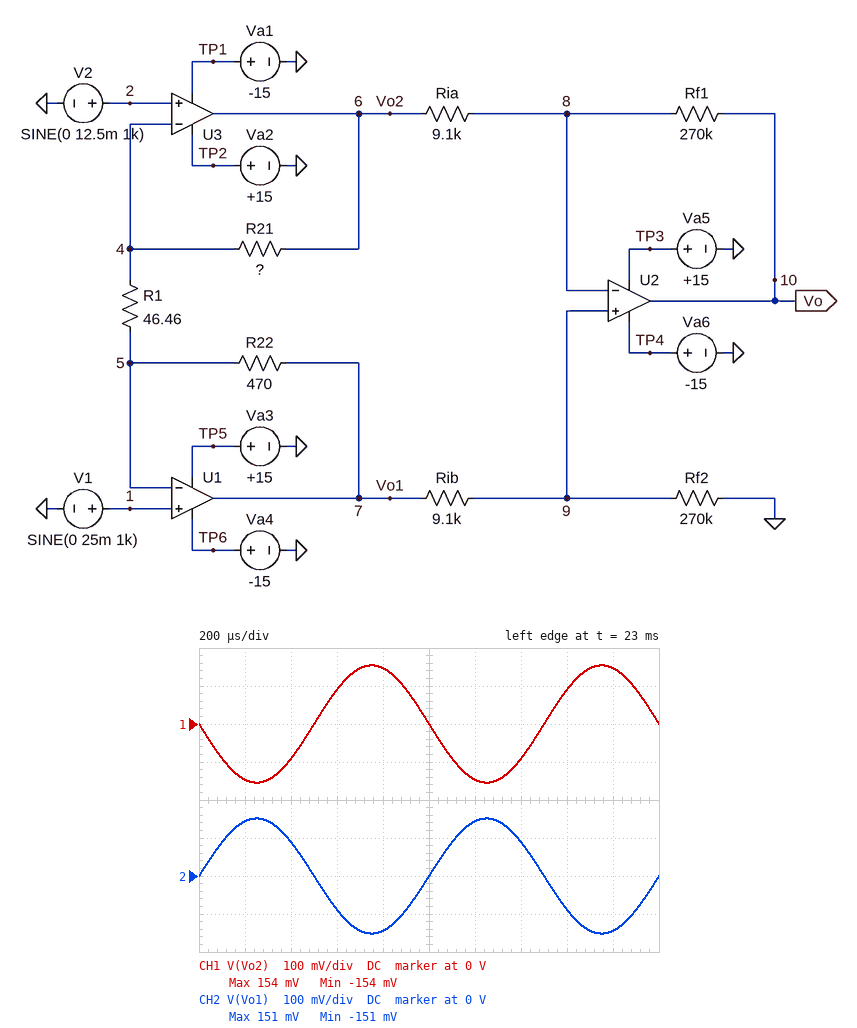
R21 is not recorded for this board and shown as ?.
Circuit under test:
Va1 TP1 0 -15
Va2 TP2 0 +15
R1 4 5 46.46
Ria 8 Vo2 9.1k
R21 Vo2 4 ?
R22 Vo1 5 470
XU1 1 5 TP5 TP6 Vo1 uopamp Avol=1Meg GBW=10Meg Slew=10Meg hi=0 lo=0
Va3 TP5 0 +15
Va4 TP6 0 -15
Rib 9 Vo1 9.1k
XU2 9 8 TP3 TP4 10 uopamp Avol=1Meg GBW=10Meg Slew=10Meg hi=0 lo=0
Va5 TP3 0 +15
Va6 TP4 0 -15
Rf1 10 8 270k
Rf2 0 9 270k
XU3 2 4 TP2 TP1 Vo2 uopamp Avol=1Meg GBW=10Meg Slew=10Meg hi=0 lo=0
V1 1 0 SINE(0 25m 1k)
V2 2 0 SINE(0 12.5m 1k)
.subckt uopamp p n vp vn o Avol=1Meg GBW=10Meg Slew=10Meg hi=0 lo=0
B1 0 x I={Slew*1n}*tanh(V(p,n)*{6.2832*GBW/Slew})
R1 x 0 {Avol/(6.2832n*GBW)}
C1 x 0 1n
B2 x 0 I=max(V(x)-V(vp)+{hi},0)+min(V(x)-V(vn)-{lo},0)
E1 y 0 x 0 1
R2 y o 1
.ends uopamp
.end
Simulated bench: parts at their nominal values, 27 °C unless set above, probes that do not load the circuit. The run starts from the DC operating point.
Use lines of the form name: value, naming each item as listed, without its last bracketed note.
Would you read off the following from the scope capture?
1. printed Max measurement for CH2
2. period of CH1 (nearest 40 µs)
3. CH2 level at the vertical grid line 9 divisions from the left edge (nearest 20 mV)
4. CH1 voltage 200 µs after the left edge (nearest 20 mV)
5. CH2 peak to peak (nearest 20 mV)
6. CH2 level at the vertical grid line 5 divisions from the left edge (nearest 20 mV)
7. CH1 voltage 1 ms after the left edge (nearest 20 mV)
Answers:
printed Max measurement for CH2: 151 mV
period of CH1: 1.00 ms
CH2 level at the vertical grid line 9 divisions from the left edge: -140 mV
CH1 voltage 200 µs after the left edge: -140 mV
CH2 peak to peak: 300 mV
CH2 level at the vertical grid line 5 divisions from the left edge: 0 V
CH1 voltage 1 ms after the left edge: 0 V
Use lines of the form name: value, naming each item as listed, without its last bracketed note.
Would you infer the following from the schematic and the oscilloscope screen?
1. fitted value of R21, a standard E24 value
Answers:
fitted value of R21, a standard E24 value: 620 Ω
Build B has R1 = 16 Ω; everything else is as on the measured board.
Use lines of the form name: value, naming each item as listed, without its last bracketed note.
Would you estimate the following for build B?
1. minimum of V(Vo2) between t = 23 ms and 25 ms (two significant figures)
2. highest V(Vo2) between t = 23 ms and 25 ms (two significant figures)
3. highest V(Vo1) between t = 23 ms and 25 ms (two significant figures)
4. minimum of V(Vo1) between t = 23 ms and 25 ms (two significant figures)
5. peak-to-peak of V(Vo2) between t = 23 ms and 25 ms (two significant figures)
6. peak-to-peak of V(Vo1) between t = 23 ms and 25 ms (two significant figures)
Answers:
minimum of V(Vo2) between t = 23 ms and 25 ms: -470 mV
highest V(Vo2) between t = 23 ms and 25 ms: 470 mV
highest V(Vo1) between t = 23 ms and 25 ms: 390 mV
minimum of V(Vo1) between t = 23 ms and 25 ms: -390 mV
peak-to-peak of V(Vo2) between t = 23 ms and 25 ms: 940 mV
peak-to-peak of V(Vo1) between t = 23 ms and 25 ms: 780 mV
